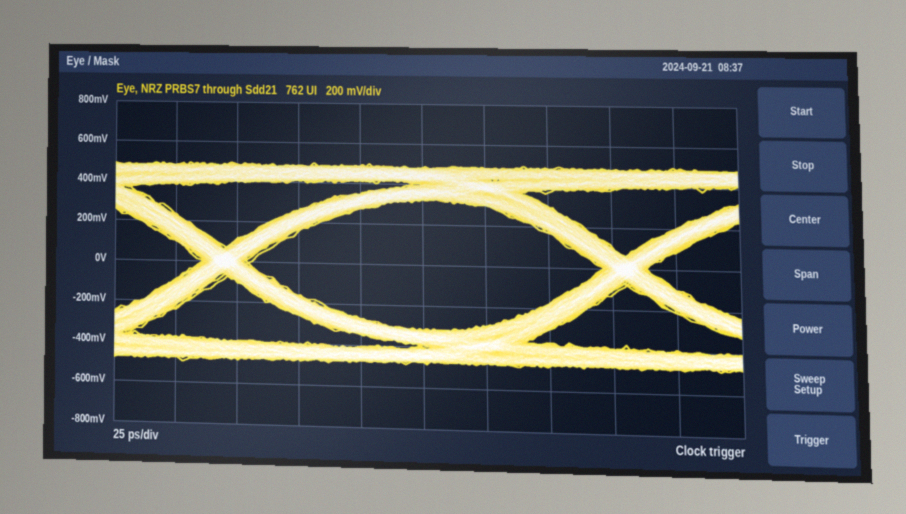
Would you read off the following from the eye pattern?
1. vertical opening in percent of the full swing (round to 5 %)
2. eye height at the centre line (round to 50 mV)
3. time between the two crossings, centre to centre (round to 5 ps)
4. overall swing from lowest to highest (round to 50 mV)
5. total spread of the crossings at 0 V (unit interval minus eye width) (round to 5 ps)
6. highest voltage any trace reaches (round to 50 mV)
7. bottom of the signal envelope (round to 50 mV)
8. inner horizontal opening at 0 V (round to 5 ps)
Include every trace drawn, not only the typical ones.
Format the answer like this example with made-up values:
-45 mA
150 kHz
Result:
65 %
650 mV
160 ps
1.00 V
20 ps
500 mV
-500 mV
140 ps
